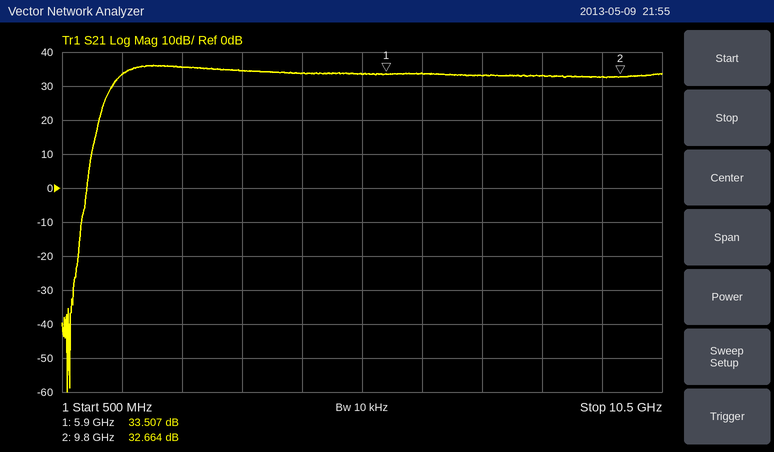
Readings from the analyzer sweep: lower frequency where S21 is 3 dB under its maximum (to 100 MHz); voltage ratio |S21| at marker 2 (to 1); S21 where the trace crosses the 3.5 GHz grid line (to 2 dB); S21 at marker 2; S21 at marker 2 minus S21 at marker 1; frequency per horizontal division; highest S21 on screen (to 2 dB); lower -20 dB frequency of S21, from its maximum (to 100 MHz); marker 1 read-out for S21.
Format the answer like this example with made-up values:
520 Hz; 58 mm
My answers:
1.5 GHz; 43; 34 dB; 32.664 dB; -0.843 dB; 1 GHz; 36 dB; 1.1 GHz; 33.507 dB
